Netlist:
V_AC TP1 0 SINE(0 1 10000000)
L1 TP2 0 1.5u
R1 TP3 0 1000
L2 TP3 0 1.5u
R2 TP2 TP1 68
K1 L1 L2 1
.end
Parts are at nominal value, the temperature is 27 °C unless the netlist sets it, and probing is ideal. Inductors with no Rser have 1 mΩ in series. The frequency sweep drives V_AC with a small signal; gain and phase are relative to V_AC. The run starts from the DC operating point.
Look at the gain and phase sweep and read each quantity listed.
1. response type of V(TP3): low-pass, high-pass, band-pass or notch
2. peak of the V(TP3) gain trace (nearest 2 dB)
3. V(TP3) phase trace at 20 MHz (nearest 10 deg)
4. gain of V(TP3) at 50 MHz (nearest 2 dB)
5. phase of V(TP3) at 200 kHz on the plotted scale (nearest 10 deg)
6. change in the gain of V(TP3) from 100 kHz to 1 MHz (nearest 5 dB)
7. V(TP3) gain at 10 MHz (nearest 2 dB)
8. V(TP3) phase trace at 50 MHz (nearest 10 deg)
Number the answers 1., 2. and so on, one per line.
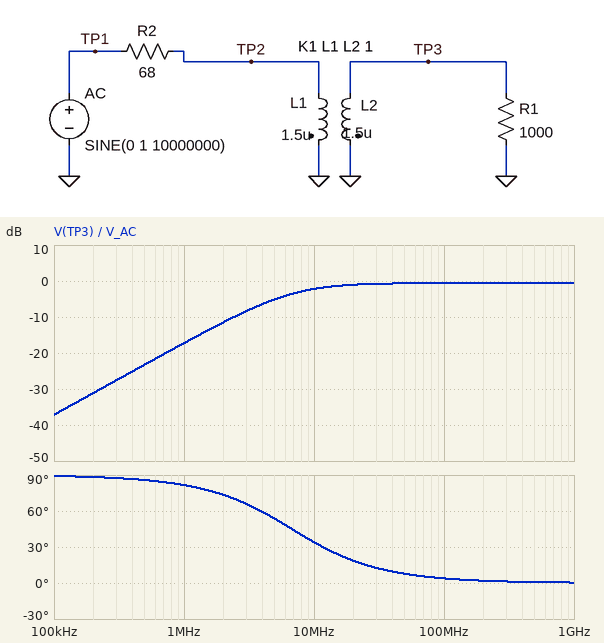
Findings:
1. high-pass
2. 0 dB
3. 20 deg
4. 0 dB
5. 90 deg
6. 20 dB
7. -2 dB
8. 10 deg
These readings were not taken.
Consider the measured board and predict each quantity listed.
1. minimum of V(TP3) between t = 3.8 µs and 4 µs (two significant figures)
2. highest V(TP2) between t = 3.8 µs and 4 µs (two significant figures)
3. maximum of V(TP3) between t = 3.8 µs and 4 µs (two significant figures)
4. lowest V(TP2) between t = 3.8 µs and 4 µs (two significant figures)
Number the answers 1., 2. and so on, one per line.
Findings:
1. -780 mV
2. 780 mV
3. 780 mV
4. -780 mV
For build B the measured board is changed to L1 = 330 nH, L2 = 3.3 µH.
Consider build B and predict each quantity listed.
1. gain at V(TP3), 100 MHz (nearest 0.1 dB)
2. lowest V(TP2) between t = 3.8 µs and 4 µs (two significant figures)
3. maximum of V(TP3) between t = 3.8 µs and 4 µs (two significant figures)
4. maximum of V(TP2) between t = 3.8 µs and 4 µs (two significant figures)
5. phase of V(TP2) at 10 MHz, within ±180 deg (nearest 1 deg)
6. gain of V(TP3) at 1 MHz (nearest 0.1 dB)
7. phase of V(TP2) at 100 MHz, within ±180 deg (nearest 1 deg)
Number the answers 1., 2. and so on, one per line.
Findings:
1. 5.3 dB
2. -270 mV
3. 860 mV
4. 270 mV
5. 63 deg
6. -20.3 dB
7. 11 deg
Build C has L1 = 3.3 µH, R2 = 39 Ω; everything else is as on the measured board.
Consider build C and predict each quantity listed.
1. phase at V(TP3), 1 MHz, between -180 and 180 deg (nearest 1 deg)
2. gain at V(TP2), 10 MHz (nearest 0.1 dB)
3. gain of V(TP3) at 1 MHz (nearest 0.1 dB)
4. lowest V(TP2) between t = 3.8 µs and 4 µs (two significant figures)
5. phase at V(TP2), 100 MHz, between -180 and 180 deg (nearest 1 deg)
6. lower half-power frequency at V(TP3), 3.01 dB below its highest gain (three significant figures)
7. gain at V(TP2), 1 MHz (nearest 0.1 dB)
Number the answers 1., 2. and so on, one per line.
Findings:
1. 62 deg
2. -0.3 dB
3. -10.0 dB
4. -970 mV
5. 1 deg
6. 1.85 MHz
7. -6.6 dB
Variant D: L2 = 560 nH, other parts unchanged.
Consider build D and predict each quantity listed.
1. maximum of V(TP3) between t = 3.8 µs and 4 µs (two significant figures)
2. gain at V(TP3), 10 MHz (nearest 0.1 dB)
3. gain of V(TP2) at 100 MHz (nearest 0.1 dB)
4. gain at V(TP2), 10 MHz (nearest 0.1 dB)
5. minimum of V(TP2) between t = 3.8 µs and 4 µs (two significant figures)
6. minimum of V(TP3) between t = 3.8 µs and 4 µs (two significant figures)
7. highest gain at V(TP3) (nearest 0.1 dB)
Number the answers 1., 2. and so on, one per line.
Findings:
1. 490 mV
2. -6.2 dB
3. -0.2 dB
4. -2.0 dB
5. -800 mV
6. -490 mV
7. -4.5 dB
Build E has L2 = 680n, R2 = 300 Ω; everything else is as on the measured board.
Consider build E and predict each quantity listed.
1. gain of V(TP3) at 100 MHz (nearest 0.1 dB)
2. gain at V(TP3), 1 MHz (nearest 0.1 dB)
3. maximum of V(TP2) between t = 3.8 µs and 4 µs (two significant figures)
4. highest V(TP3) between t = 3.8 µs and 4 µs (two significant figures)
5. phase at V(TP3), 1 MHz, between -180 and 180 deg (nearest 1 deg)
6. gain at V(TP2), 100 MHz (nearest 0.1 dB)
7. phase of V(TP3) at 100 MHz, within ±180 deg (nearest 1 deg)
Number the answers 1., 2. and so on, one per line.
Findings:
1. -4.9 dB
2. -33.5 dB
3. 300 mV
4. 200 mV
5. 88 deg
6. -1.4 dB
7. 16 deg
